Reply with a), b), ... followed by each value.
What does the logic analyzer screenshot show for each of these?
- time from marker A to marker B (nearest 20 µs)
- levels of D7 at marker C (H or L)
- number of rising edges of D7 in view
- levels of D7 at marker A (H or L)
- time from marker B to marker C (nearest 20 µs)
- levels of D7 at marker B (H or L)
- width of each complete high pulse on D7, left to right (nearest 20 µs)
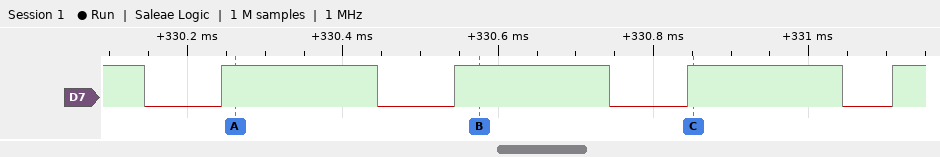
a) 320 µs
b) D7=H
c) 4
d) D7=H
e) 280 µs
f) D7=H
g) 200 µs, 200 µs, 200 µs
